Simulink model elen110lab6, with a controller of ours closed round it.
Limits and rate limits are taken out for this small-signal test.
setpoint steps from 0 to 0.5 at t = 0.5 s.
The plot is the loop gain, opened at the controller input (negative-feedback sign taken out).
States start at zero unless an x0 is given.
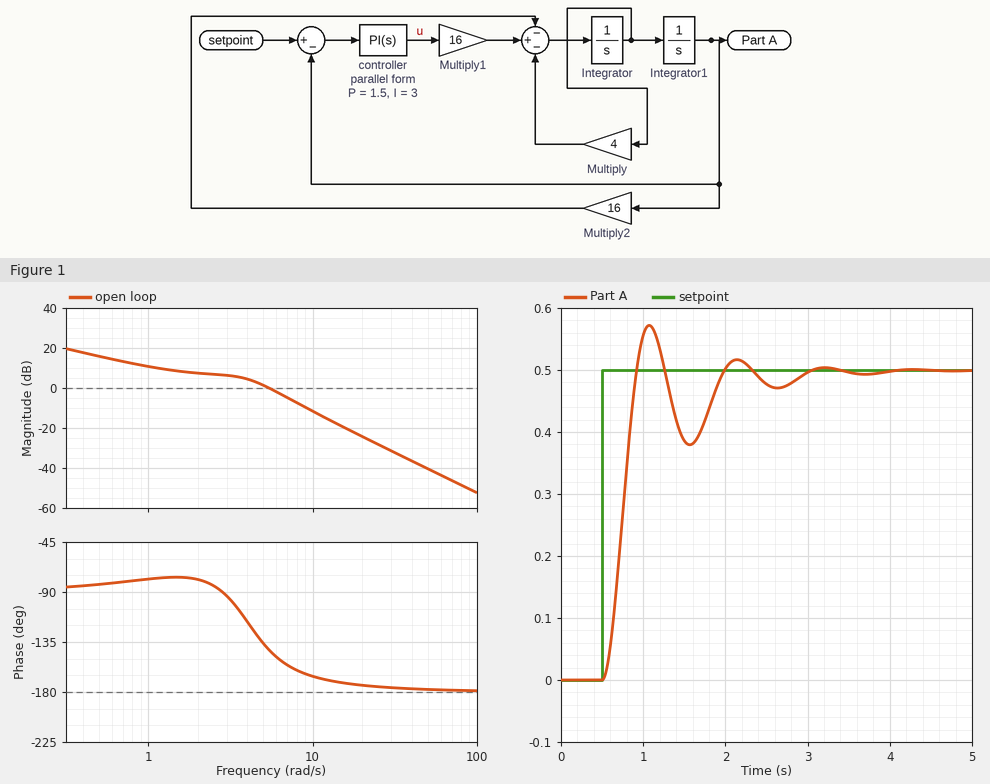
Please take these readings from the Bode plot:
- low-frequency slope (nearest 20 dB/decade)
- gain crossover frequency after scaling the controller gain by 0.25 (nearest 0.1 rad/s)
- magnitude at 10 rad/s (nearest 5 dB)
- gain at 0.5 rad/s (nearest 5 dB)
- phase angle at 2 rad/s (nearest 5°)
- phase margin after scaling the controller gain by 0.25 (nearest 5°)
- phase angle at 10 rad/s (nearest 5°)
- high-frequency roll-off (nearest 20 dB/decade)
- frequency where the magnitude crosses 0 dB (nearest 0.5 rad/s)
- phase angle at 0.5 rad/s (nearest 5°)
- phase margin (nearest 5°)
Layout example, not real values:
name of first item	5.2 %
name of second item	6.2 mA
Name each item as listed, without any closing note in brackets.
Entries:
low-frequency slope	-20 dB/decade
gain crossover frequency after scaling the controller gain by 0.25	0.8 rad/s
magnitude at 10 rad/s	-10 dB
gain at 0.5 rad/s	15 dB
phase angle at 2 rad/s	-80°
phase margin after scaling the controller gain by 0.25	100°
phase angle at 10 rad/s	-165°
high-frequency roll-off	-40 dB/decade
frequency where the magnitude crosses 0 dB	5.5 rad/s
phase angle at 0.5 rad/s	-85°
phase margin	40°
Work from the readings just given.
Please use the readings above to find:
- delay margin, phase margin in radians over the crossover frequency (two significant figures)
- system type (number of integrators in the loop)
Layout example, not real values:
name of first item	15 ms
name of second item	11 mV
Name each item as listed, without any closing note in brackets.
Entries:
delay margin, phase margin in radians over the crossover frequency	0.13 s
system type	1
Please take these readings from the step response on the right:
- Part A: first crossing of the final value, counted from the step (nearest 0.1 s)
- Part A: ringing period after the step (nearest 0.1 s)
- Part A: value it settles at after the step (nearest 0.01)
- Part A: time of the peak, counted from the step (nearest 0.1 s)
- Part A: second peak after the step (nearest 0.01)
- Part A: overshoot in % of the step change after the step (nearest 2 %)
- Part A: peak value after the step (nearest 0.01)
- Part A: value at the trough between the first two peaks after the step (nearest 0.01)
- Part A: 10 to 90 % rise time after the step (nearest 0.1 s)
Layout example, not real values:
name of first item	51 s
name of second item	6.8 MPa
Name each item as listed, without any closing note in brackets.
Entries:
Part A: first crossing of the final value, counted from the step	0.4 s
Part A: ringing period after the step	1.1 s
Part A: value it settles at after the step	0.50
Part A: time of the peak, counted from the step	0.6 s
Part A: second peak after the step	0.52
Part A: overshoot in % of the step change after the step	14 %
Part A: peak value after the step	0.57
Part A: value at the trough between the first two peaks after the step	0.38
Part A: 10 to 90 % rise time after the step	0.3 s
